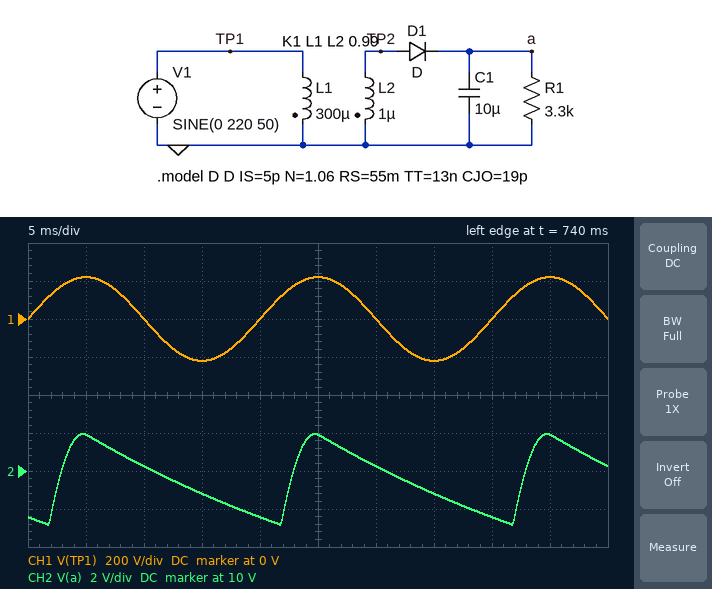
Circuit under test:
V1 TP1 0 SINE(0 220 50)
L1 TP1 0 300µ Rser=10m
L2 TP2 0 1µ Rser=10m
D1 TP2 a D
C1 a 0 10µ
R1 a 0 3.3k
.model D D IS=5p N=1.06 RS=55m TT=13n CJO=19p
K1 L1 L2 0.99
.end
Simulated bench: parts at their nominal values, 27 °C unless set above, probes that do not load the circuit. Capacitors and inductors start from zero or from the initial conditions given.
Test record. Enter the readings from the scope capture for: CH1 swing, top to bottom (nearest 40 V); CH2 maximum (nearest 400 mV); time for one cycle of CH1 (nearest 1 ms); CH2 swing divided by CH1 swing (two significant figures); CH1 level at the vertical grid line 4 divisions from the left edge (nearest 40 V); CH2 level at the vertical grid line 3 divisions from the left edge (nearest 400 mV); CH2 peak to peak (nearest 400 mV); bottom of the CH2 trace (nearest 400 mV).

440 V
12.0 V
20 ms
0.011
0 V
8.8 V
4.8 V
7.2 V
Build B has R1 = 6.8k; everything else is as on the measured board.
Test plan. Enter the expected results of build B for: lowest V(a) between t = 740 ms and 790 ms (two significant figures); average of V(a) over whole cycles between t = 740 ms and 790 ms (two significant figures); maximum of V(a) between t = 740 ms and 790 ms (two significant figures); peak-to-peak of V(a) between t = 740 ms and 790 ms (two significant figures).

9.2 V
11 V
12 V
2.7 V
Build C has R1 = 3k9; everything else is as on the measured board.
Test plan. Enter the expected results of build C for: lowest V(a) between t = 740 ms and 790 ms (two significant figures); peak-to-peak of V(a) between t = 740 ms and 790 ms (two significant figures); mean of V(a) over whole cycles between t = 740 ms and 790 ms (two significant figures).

7.7 V
4.2 V
9.8 V
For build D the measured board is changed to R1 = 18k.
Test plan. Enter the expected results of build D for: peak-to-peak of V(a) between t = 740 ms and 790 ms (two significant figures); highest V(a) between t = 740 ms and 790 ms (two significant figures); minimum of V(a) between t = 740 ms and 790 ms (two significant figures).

1.2 V
12 V
11 V
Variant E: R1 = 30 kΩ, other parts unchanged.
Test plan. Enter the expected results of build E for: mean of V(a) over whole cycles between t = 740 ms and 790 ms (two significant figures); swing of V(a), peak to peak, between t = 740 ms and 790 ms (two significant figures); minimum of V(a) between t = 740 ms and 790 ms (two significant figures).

12 V
720 mV
11 V
